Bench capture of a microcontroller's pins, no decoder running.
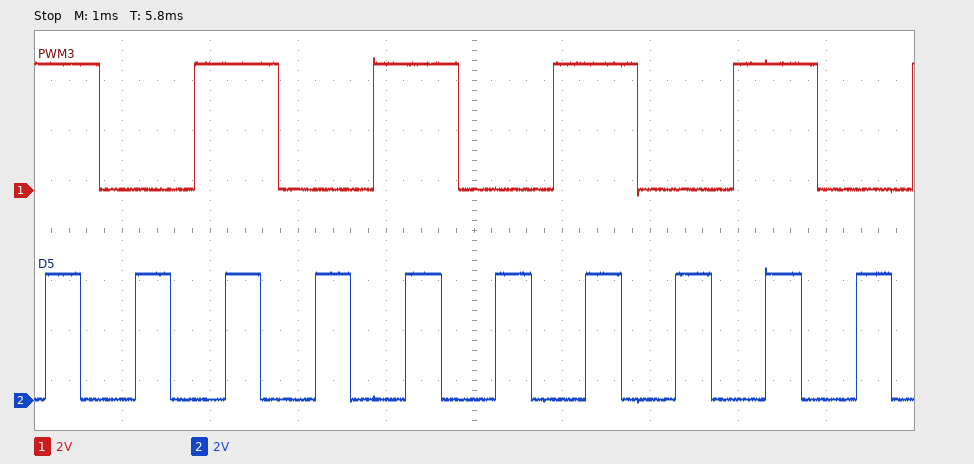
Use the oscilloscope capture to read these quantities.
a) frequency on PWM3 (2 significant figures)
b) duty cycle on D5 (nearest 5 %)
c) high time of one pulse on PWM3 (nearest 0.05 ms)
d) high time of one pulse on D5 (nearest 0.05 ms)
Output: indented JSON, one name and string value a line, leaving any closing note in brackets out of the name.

{
  "frequency on PWM3": "490 Hz",
  "duty cycle on D5": "40 %",
  "high time of one pulse on PWM3": "0.95 ms",
  "high time of one pulse on D5": "0.40 ms"
}
